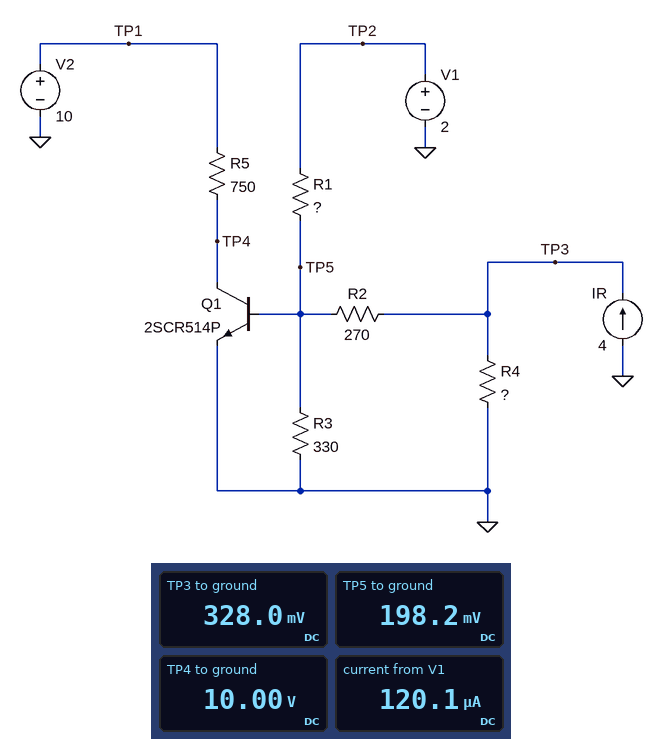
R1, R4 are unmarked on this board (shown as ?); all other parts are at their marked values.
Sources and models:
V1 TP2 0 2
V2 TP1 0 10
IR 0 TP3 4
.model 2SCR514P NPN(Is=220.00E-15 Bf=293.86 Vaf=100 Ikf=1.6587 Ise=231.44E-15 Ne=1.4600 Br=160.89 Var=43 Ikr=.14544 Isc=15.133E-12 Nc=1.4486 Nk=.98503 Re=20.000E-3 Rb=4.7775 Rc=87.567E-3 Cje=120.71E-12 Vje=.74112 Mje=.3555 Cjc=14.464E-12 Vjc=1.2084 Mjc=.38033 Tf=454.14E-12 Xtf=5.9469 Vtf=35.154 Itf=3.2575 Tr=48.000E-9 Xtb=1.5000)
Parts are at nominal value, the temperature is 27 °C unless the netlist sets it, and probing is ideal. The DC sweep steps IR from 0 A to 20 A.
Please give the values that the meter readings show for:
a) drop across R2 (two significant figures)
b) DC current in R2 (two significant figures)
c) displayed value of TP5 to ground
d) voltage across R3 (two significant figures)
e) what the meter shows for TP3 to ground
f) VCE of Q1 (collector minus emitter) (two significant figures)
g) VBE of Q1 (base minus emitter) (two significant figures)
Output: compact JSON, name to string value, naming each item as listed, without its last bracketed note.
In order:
{"drop across R2": "130 mV", "DC current in R2": "480 µA", "displayed value of TP5 to ground": "198.2 mV", "voltage across R3": "200 mV", "what the meter shows for TP3 to ground": "328.0 mV", "VCE of Q1 (collector minus emitter)": "10 V", "VBE of Q1 (base minus emitter)": "200 mV"}
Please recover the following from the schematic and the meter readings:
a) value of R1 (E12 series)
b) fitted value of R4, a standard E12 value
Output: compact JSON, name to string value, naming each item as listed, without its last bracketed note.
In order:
{"value of R1": "15 kΩ", "fitted value of R4, a standard E12 value": "0.082 Ω"}
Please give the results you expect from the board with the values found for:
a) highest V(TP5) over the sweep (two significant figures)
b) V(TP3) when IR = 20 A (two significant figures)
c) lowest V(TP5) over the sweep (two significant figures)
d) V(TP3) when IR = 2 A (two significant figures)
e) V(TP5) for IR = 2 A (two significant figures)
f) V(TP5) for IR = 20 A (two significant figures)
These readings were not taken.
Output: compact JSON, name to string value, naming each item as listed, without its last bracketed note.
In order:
{"highest V(TP5) over the sweep": "690 mV", "V(TP3) when IR = 20 A": "1.6 V", "lowest V(TP5) over the sweep": "20 mV", "V(TP3) when IR = 2 A": "160 mV", "V(TP5) for IR = 2 A": "110 mV", "V(TP5) for IR = 20 A": "690 mV"}
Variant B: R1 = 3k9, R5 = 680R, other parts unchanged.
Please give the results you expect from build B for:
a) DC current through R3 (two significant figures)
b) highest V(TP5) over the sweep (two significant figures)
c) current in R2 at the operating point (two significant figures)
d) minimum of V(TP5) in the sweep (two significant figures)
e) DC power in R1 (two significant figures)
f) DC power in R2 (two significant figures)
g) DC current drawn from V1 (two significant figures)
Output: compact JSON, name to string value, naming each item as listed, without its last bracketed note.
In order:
{"DC current through R3": "750 µA", "highest V(TP5) over the sweep": "700 mV", "current in R2 at the operating point": "300 µA", "minimum of V(TP5) in the sweep": "73 mV", "DC power in R1": "790 µW", "DC power in R2": "24 µW", "DC current drawn from V1": "450 µA"}
